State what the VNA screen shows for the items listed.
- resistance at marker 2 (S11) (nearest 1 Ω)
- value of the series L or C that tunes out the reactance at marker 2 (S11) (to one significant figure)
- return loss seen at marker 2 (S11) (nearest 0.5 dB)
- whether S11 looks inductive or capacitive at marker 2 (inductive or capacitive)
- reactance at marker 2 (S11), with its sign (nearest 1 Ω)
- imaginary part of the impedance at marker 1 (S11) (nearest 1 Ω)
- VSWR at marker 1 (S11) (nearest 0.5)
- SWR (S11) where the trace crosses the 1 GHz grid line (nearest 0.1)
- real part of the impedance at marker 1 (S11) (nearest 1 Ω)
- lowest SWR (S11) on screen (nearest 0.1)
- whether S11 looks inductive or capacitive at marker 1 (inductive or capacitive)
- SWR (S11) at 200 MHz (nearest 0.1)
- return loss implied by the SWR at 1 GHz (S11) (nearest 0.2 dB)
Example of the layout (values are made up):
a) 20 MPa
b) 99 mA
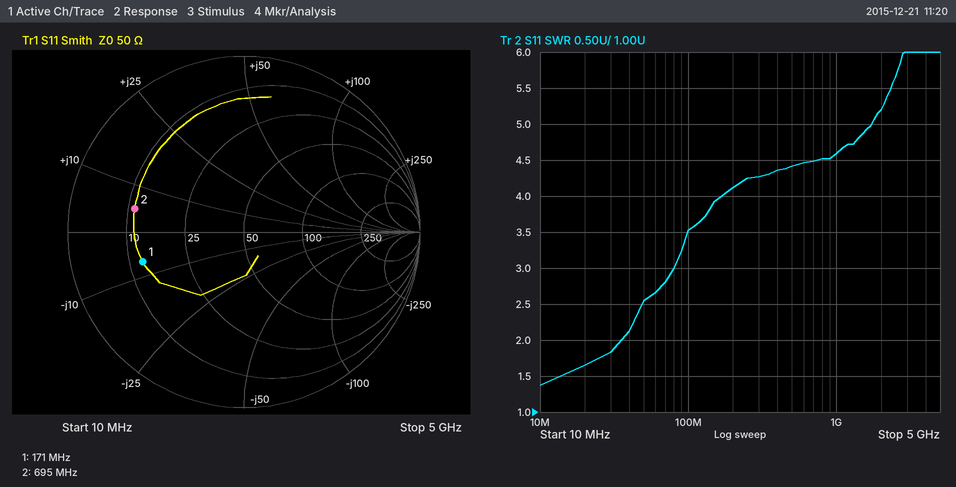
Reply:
a) 11 Ω
b) 50 pF
c) 4.0 dB
d) inductive
e) +5 Ω
f) -7 Ω
g) 4.0
h) 4.6
i) 13 Ω
j) 1.4
k) capacitive
l) 4.1
m) 3.8 dB
